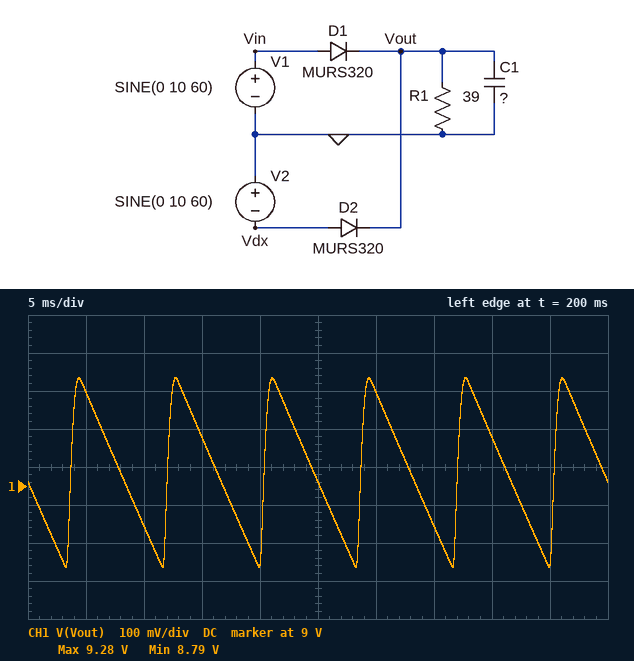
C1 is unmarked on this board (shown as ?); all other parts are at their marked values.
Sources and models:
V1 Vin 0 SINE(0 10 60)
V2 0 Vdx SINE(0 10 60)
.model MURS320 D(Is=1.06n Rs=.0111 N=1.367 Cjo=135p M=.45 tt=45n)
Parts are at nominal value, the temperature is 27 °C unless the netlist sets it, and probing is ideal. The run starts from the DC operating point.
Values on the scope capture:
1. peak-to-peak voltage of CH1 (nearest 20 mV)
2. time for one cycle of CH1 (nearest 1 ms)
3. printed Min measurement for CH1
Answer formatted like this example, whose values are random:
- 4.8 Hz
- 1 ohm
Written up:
- 500 mV
- 8 ms
- 8.79 V
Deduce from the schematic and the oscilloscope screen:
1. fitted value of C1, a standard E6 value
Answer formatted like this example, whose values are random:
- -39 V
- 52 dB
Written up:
- 3.3 mF
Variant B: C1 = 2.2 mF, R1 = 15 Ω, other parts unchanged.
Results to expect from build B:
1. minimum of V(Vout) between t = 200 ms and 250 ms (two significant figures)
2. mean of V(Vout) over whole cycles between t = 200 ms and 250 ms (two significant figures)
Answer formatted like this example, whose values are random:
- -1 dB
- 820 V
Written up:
- 7.6 V
- 8.5 V
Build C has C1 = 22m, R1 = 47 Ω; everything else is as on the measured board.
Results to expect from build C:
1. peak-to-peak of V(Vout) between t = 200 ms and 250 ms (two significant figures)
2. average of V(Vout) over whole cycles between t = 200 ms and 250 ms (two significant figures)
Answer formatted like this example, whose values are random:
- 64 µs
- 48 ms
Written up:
- 65 mV
- 9.2 V
